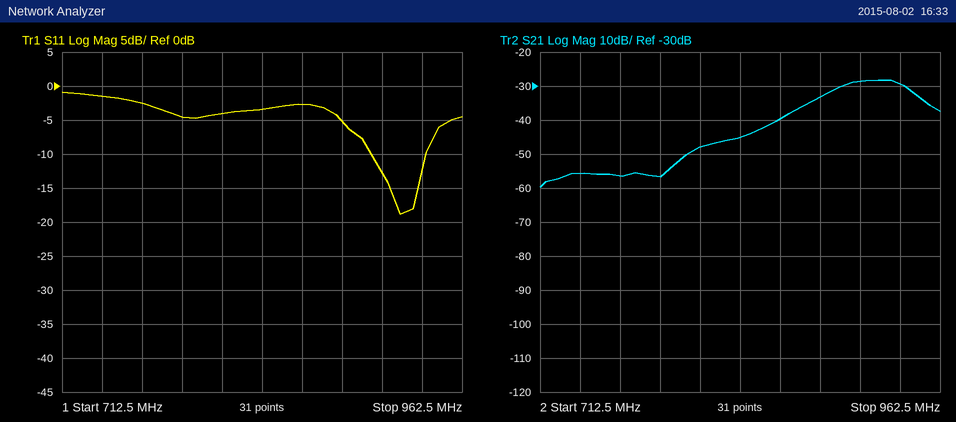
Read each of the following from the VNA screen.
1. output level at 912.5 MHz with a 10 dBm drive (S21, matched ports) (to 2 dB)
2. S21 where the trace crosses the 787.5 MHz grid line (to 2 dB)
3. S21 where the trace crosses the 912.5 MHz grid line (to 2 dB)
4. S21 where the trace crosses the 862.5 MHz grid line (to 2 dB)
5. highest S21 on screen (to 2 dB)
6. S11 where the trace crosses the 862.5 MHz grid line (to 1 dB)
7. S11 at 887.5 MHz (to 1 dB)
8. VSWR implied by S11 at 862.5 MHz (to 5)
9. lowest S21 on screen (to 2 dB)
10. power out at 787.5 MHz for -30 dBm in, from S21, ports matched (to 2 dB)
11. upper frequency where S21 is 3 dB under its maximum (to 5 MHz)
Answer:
-18 dBm
-56 dB
-28 dB
-40 dB
-28 dB
-3 dB
-5 dB
5
-60 dB
-86 dBm
945 MHz
